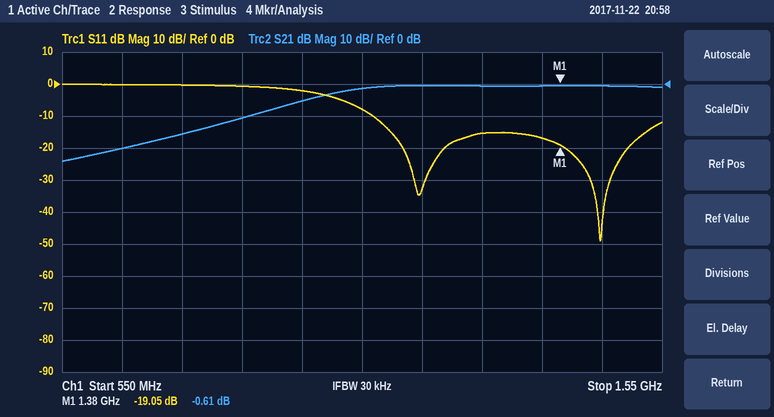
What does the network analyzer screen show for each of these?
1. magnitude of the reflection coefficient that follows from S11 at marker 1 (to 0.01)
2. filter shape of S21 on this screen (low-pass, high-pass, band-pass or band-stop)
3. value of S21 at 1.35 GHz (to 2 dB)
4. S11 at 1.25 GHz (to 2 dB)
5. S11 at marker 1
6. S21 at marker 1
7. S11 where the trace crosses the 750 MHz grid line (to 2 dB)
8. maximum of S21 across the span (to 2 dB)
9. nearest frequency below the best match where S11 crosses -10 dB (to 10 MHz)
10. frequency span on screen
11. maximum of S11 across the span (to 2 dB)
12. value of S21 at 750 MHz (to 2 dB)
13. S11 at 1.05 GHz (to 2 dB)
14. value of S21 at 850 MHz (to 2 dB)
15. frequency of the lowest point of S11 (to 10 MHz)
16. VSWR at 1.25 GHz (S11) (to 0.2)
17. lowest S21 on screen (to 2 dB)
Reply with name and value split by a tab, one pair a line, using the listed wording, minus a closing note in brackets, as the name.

magnitude of the reflection coefficient that follows from S11 at marker 1	0.11
filter shape of S21 on this screen	high-pass
value of S21 at 1.35 GHz	0 dB
S11 at 1.25 GHz	-16 dB
S11 at marker 1	-19.05 dB
S21 at marker 1	-0.61 dB
S11 where the trace crosses the 750 MHz grid line	0 dB
maximum of S21 across the span	0 dB
nearest frequency below the best match where S11 crosses -10 dB	1.07 GHz
frequency span on screen	1 GHz
maximum of S11 across the span	0 dB
value of S21 at 750 MHz	-16 dB
S11 at 1.05 GHz	-8 dB
value of S21 at 850 MHz	-10 dB
frequency of the lowest point of S11	1.45 GHz
VSWR at 1.25 GHz (S11)	1.4
lowest S21 on screen	-24 dB
